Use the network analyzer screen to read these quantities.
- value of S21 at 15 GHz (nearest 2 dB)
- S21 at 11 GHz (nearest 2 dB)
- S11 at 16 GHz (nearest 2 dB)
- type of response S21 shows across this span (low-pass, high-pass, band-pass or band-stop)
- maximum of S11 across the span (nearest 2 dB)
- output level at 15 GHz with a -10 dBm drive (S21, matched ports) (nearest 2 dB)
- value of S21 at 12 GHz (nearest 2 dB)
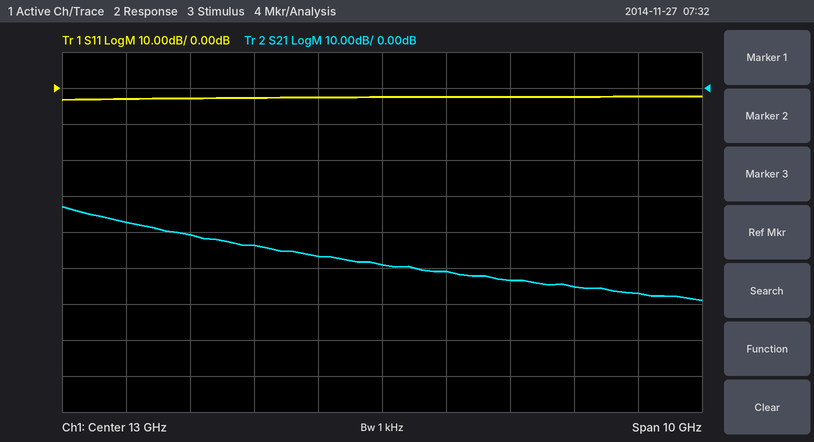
-54 dB
-44 dB
-2 dB
low-pass
-2 dB
-64 dBm
-46 dB
